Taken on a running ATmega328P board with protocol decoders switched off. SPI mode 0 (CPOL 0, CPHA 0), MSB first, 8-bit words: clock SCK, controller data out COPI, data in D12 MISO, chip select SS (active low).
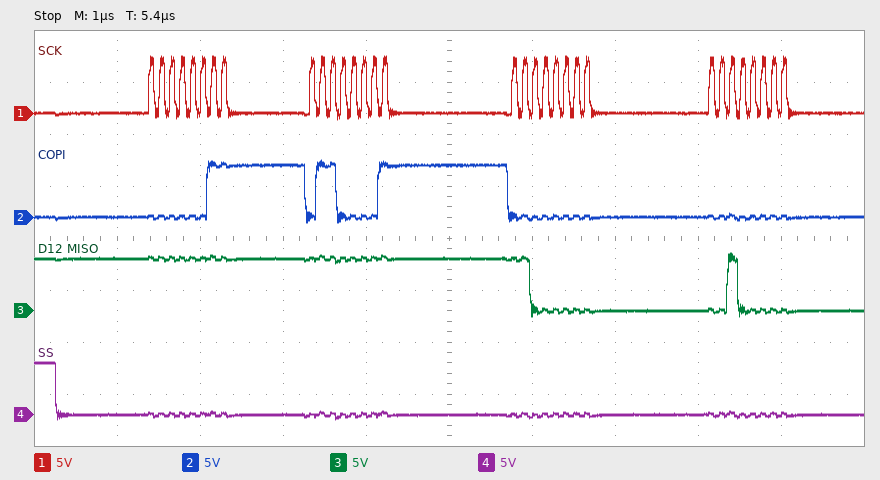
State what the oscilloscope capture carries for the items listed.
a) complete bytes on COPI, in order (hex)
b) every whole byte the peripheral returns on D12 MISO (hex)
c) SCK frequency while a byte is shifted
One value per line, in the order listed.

0x03 0x61 0x00 0x00
0xFF 0xFF 0xC0 0x20
8 MHz
